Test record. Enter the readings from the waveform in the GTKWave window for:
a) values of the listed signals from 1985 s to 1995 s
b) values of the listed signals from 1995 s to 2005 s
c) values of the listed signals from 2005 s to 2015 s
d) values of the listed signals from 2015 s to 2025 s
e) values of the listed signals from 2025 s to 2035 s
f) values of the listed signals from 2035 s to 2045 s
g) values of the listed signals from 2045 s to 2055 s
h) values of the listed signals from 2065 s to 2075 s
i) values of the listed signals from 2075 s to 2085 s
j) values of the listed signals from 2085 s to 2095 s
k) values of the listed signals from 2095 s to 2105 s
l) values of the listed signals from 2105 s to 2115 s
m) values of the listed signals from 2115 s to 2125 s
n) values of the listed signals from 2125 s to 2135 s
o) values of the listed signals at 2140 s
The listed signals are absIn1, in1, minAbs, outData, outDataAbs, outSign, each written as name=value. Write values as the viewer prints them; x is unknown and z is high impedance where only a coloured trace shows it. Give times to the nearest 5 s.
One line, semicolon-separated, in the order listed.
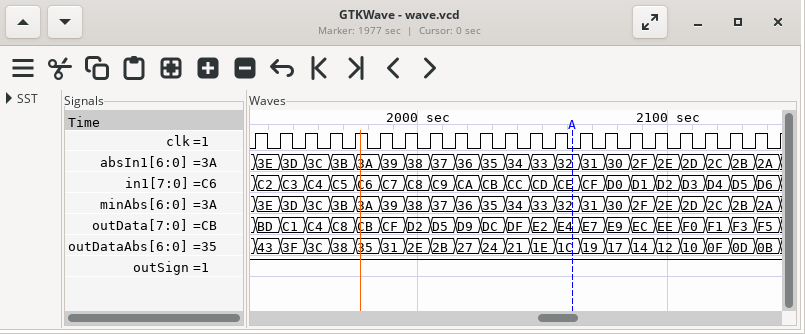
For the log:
absIn1=39, in1=C7, minAbs=39, outData=CF, outDataAbs=31, outSign=1; absIn1=38, in1=C8, minAbs=38, outData=D2, outDataAbs=2E, outSign=1; absIn1=37, in1=C9, minAbs=37, outData=D5, outDataAbs=2B, outSign=1; absIn1=36, in1=CA, minAbs=36, outData=D9, outDataAbs=27, outSign=1; absIn1=35, in1=CB, minAbs=35, outData=DC, outDataAbs=24, outSign=1; absIn1=34, in1=CC, minAbs=34, outData=DF, outDataAbs=21, outSign=1; absIn1=33, in1=CD, minAbs=33, outData=E2, outDataAbs=1E, outSign=1; absIn1=31, in1=CF, minAbs=31, outData=E7, outDataAbs=19, outSign=1; absIn1=30, in1=D0, minAbs=30, outData=E9, outDataAbs=17, outSign=1; absIn1=2F, in1=D1, minAbs=2F, outData=EC, outDataAbs=14, outSign=1; absIn1=2E, in1=D2, minAbs=2E, outData=EE, outDataAbs=12, outSign=1; absIn1=2D, in1=D3, minAbs=2D, outData=F0, outDataAbs=10, outSign=1; absIn1=2C, in1=D4, minAbs=2C, outData=F1, outDataAbs=0F, outSign=1; absIn1=2B, in1=D5, minAbs=2B, outData=F3, outDataAbs=0D, outSign=1; absIn1=2A, in1=D6, minAbs=2A, outData=F5, outDataAbs=0B, outSign=1
